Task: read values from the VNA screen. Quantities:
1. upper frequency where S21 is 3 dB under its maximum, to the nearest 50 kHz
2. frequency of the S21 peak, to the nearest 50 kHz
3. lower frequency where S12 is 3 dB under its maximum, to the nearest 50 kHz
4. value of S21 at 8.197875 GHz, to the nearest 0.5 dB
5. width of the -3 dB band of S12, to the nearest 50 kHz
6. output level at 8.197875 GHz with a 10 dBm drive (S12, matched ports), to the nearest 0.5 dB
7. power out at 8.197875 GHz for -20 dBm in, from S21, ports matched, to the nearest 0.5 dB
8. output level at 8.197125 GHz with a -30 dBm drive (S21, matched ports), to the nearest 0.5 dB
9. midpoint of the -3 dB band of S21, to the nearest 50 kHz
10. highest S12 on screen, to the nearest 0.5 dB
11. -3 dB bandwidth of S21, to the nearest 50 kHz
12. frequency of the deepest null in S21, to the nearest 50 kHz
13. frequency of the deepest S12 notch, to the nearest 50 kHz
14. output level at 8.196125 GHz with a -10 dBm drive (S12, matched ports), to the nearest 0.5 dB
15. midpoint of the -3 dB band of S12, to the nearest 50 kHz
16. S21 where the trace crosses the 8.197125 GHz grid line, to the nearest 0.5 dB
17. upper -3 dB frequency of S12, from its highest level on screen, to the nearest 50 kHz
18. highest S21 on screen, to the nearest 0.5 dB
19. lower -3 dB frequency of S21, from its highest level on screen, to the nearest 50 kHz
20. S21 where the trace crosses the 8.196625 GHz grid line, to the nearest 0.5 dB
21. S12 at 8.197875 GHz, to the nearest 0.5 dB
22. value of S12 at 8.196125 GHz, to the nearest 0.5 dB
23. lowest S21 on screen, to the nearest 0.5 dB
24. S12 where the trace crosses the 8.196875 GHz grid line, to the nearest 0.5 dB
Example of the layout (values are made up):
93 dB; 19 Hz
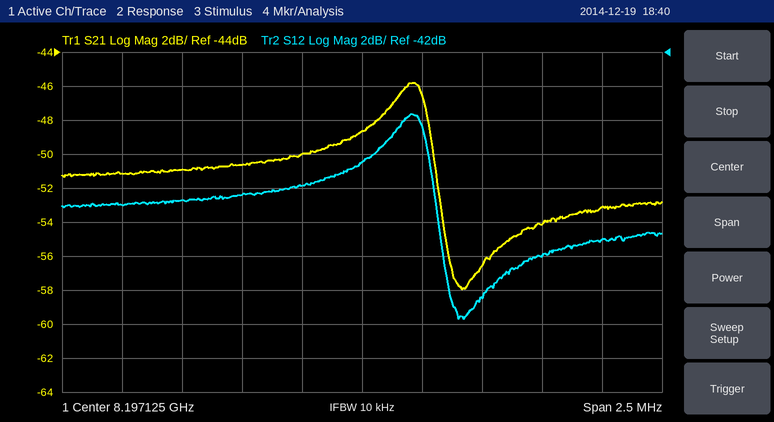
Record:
8.19740 GHz; 8.19735 GHz; 8.19710 GHz; -54.0 dB; 300 kHz; -44.0 dBm; -74.0 dBm; -78.5 dBm; 8.19725 GHz; -45.5 dB; 300 kHz; 8.19755 GHz; 8.19755 GHz; -61.0 dBm; 8.19725 GHz; -48.5 dB; 8.19740 GHz; -46.0 dB; 8.19710 GHz; -50.5 dB; -54.0 dB; -51.0 dB; -58.0 dB; -50.0 dB
